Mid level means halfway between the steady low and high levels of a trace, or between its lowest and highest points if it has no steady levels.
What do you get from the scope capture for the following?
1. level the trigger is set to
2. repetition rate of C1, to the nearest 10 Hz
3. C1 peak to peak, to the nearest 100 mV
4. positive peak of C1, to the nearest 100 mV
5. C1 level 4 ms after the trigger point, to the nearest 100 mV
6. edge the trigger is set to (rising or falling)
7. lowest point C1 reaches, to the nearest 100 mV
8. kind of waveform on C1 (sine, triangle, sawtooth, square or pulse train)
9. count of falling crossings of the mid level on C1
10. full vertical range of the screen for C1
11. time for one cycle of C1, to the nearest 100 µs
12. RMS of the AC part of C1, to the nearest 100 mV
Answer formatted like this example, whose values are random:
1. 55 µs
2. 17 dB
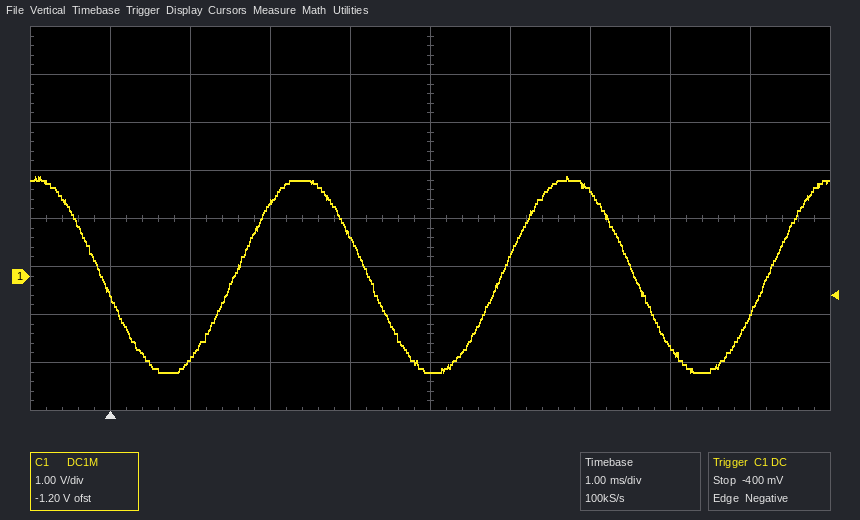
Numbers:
1. -400 mV
2. 300 Hz
3. 4.1 V
4. 2.1 V
5. -2.0 V
6. falling
7. -2.0 V
8. sine
9. 3
10. 8 V
11. 3.3 ms
12. 1.4 V
